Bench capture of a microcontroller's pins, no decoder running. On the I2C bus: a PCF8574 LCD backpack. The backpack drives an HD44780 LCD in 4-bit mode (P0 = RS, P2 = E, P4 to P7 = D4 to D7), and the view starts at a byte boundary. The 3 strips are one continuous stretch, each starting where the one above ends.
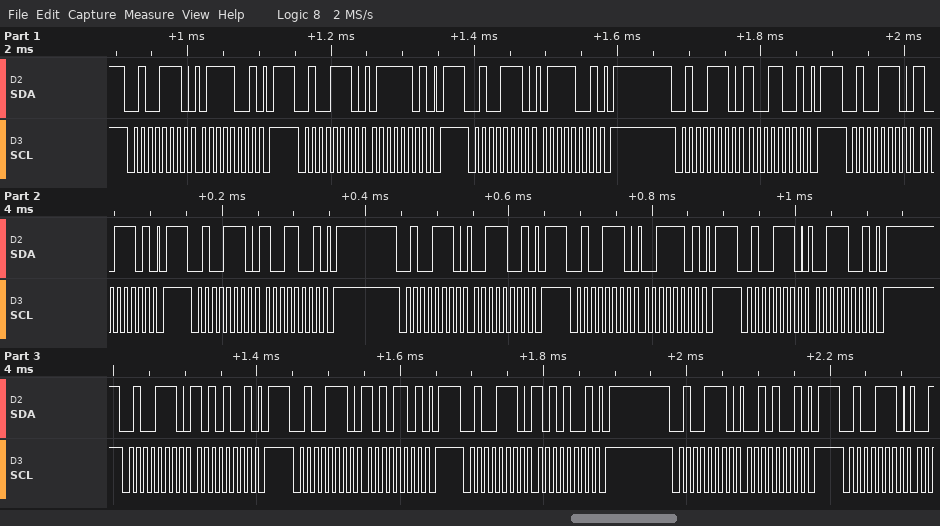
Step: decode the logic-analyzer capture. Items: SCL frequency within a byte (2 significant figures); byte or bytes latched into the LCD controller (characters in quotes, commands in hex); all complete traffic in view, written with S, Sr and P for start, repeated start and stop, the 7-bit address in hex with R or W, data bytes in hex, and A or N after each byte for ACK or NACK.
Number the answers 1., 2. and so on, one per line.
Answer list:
1. 100 kHz
2. 'y' ':'
3. S 27W A 79 A P S 27W A 7D A P S 27W A 79 A P S 27W A 99 A P S 27W A 9D A P S 27W A 99 A P S 27W A 39 A P S 27W A 3D A P S 27W A 39 A P S 27W A A9 A P S 27W A AD A P S 27W A A9 A P S 27W A 29 A P S 27W A
